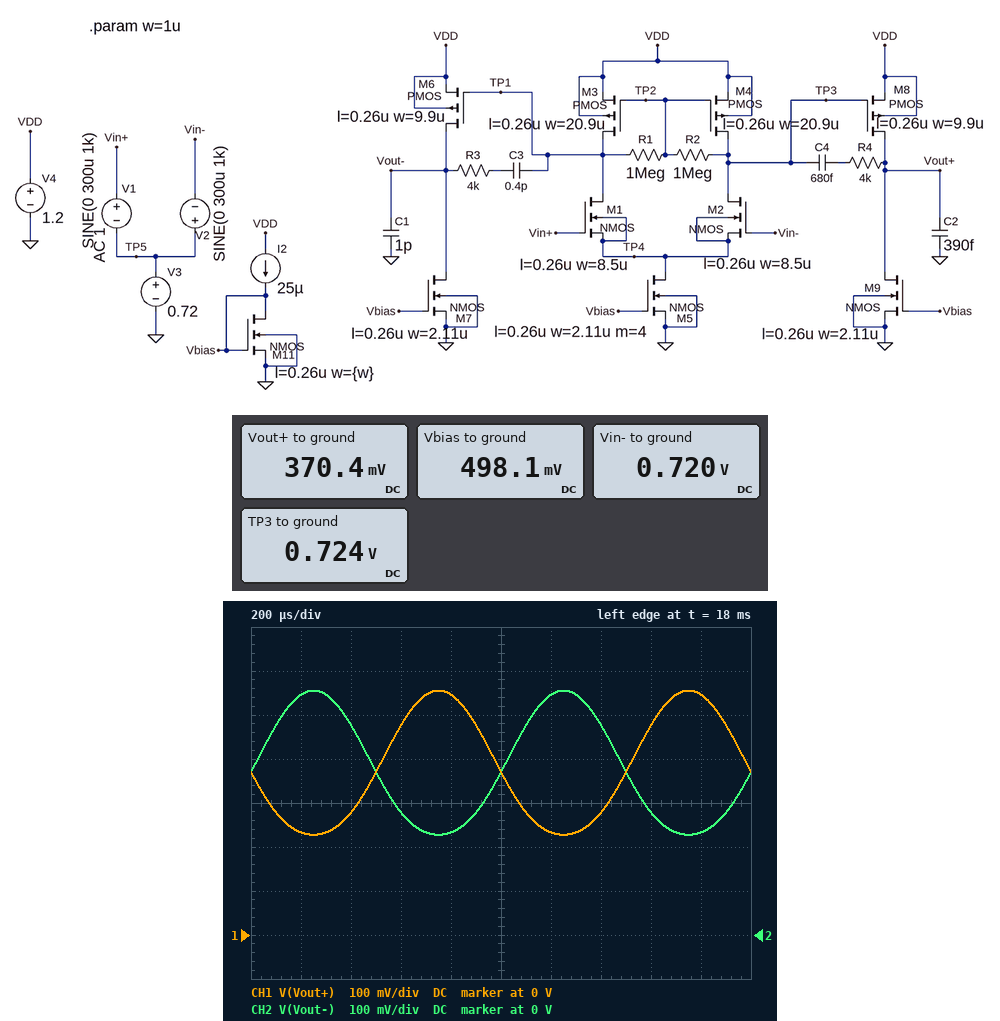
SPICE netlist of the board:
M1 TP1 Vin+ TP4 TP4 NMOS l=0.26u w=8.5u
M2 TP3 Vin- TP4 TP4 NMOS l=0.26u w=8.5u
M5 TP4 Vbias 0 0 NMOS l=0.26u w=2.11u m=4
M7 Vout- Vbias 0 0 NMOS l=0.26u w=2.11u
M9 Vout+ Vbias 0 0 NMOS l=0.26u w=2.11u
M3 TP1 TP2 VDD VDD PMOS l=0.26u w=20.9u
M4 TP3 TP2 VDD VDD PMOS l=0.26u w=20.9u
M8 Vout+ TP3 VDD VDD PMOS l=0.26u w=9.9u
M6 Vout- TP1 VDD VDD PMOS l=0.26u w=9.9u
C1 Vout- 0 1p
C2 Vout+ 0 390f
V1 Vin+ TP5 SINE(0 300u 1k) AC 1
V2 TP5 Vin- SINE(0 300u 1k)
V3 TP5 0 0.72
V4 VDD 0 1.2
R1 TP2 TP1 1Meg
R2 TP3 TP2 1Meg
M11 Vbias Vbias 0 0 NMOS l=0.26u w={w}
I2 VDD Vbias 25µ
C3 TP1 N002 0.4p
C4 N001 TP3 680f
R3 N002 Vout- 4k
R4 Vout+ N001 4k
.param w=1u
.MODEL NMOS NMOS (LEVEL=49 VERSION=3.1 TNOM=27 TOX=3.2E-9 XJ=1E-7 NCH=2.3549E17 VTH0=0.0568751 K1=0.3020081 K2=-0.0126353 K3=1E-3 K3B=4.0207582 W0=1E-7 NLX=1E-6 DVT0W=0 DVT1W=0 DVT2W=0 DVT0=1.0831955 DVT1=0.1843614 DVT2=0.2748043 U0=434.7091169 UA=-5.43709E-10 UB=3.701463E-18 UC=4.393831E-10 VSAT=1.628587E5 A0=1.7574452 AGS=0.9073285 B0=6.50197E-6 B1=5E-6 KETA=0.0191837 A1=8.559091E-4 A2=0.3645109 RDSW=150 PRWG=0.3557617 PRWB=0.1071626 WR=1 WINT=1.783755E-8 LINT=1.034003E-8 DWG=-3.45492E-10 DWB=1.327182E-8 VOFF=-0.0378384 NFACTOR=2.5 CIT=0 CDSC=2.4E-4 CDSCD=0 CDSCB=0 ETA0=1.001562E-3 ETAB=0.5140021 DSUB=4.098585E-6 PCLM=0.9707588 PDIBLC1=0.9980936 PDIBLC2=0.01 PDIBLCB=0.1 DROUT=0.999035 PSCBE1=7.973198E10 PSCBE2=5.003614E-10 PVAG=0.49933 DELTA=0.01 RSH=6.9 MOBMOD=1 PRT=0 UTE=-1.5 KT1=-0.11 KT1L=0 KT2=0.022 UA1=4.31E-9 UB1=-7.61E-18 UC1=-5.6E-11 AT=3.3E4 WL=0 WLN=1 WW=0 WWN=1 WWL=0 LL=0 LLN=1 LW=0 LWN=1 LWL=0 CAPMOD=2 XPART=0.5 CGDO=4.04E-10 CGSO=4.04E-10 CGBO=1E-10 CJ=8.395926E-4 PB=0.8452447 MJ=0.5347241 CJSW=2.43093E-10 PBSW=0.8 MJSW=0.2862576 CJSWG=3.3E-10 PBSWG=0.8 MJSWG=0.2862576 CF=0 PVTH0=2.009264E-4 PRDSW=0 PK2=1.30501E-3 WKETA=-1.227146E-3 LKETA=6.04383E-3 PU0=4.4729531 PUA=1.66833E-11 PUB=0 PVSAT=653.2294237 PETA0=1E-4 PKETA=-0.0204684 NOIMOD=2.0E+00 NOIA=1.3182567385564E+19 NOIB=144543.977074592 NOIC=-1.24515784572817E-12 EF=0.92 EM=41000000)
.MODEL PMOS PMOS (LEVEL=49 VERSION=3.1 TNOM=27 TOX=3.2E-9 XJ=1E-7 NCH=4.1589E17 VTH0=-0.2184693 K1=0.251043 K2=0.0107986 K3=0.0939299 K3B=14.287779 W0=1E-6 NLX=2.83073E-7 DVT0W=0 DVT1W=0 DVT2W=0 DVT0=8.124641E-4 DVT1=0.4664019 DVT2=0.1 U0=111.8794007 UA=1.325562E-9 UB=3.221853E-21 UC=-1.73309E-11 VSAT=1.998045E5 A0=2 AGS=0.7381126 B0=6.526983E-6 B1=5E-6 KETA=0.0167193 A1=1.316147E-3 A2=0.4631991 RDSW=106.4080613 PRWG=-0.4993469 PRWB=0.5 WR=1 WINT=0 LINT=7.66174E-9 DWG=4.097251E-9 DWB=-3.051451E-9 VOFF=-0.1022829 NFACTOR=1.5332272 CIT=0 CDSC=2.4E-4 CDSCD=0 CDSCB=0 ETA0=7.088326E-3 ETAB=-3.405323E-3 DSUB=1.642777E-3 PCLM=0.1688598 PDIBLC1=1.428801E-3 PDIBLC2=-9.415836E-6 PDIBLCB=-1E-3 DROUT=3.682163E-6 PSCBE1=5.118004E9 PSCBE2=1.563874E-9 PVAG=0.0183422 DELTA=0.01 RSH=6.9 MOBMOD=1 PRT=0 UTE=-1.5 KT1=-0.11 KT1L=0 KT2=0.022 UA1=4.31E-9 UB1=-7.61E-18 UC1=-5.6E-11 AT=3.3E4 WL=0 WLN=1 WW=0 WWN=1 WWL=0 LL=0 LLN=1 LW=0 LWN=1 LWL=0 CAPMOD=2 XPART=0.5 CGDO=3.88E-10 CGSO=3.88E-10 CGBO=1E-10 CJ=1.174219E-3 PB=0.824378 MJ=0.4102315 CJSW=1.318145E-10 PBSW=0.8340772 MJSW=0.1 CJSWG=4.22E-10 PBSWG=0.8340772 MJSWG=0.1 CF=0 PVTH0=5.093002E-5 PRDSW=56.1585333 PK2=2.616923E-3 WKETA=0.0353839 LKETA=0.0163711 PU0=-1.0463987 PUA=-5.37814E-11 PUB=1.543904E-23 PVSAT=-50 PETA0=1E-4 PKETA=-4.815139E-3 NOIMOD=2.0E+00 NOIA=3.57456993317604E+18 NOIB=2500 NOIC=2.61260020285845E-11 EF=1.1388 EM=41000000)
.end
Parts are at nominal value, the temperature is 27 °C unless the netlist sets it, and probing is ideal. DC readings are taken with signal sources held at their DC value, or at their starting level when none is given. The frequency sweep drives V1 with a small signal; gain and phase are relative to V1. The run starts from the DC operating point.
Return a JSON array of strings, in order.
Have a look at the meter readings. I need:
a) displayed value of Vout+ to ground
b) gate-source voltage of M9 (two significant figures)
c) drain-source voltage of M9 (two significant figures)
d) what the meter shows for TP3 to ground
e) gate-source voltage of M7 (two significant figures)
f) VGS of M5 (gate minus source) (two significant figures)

["370.4 mV", "500 mV", "370 mV", "0.724 V", "500 mV", "500 mV"]
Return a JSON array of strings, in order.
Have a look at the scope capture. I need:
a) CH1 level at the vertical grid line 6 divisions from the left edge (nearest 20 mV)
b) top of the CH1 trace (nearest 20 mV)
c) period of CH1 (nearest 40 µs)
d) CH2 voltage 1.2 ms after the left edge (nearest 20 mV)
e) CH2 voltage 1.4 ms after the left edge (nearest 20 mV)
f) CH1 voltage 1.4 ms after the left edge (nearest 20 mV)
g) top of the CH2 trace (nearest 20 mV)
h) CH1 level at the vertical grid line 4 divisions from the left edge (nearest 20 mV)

["240 mV", "560 mV", "1.00 ms", "540 mV", "480 mV", "280 mV", "560 mV", "540 mV"]
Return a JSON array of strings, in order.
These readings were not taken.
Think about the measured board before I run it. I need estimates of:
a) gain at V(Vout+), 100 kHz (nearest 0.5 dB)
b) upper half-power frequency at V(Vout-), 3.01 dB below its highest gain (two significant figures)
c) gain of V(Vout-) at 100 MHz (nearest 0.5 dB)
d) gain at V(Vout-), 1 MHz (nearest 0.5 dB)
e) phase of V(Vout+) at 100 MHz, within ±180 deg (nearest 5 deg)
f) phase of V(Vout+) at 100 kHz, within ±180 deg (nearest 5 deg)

["49.0 dB", "650 kHz", "5.0 dB", "44.0 dB", "100 deg", "170 deg"]
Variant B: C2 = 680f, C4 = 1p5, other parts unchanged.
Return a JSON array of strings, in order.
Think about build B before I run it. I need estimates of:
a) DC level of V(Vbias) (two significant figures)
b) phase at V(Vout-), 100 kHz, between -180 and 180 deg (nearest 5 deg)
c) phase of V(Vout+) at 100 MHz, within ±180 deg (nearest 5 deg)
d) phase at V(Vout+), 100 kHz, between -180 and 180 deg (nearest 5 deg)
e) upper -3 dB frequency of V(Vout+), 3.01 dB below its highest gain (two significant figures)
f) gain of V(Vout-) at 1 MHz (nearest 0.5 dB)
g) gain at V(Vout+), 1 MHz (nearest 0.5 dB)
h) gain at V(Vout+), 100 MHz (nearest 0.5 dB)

["500 mV", "-15 deg", "105 deg", "165 deg", "370 kHz", "41.0 dB", "40.0 dB", "2.5 dB"]
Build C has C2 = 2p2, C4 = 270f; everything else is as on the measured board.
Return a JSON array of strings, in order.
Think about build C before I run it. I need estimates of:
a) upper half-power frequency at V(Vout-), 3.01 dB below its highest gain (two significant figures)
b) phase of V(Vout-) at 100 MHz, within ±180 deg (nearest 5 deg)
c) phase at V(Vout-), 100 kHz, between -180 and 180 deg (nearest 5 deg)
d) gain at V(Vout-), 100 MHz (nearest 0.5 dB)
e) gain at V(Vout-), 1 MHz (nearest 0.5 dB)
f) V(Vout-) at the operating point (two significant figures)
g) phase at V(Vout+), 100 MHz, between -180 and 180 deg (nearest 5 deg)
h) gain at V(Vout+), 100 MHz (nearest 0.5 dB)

["900 kHz", "-115 deg", "-5 deg", "5.5 dB", "45.5 dB", "370 mV", "50 deg", "2.0 dB"]
